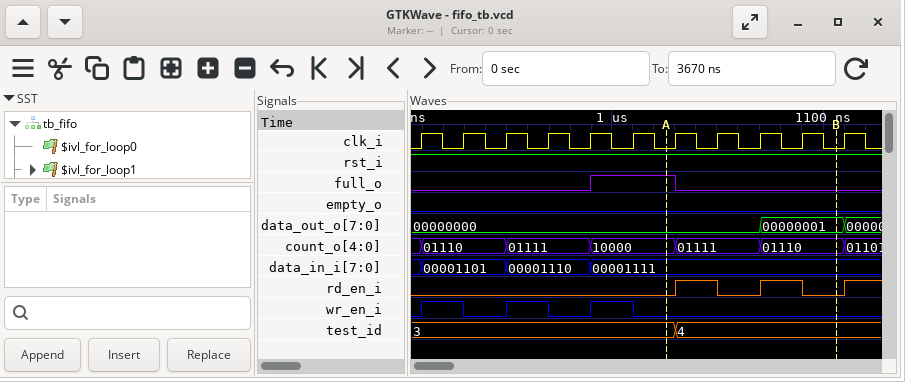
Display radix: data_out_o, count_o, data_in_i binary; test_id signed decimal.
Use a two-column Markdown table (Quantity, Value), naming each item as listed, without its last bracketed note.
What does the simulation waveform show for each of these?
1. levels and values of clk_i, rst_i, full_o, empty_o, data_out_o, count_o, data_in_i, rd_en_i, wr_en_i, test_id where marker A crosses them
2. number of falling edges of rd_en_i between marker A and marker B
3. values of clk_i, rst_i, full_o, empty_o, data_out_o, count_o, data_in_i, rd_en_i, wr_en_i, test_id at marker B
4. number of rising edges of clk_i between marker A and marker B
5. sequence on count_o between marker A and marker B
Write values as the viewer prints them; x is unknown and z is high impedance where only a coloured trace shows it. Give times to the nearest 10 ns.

| Quantity | Value |
|---|---|
| levels and values of clk_i, rst_i, full_o, empty_o, data_out_o, count_o, data_in_i, rd_en_i, wr_en_i, test_id where marker A crosses them | clk_i=0, rst_i=1, full_o=1, empty_o=0, data_out_o=00000000, count_o=10000, data_in_i=00001111, rd_en_i=0, wr_en_i=0, test_id=3 |
| number of falling edges of rd_en_i between marker A and marker B | 2 |
| values of clk_i, rst_i, full_o, empty_o, data_out_o, count_o, data_in_i, rd_en_i, wr_en_i, test_id at marker B | clk_i=0, rst_i=1, full_o=0, empty_o=0, data_out_o=00000001, count_o=01110, data_in_i=00001111, rd_en_i=0, wr_en_i=0, test_id=4 |
| number of rising edges of clk_i between marker A and marker B | 4 |
| sequence on count_o between marker A and marker B | 10000, 01111, 01110 |
